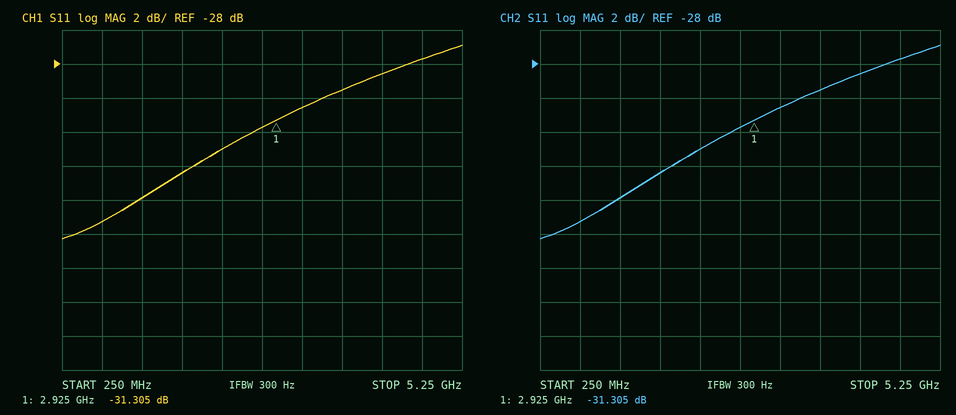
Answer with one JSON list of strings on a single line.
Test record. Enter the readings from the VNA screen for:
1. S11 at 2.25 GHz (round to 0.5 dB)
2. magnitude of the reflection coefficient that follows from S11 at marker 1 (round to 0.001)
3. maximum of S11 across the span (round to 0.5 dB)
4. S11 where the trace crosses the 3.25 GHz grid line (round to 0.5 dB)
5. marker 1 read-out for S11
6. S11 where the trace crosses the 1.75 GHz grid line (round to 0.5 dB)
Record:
["-33.0 dB", "0.027", "-27.0 dB", "-30.5 dB", "-31.305 dB", "-34.5 dB"]
